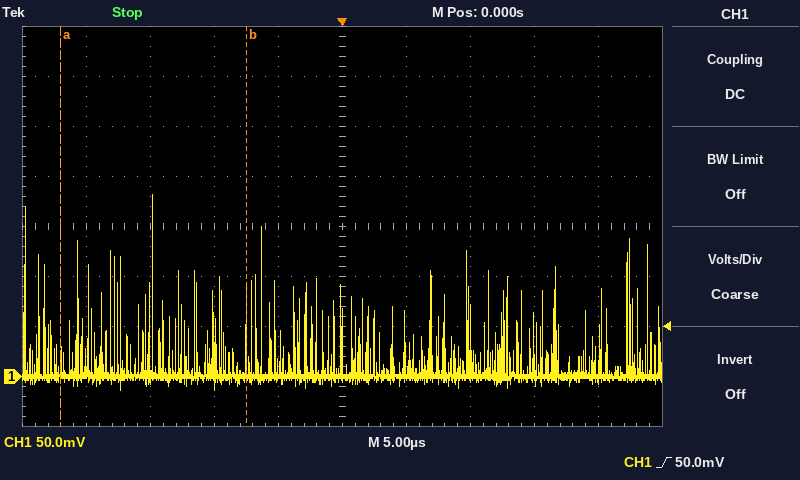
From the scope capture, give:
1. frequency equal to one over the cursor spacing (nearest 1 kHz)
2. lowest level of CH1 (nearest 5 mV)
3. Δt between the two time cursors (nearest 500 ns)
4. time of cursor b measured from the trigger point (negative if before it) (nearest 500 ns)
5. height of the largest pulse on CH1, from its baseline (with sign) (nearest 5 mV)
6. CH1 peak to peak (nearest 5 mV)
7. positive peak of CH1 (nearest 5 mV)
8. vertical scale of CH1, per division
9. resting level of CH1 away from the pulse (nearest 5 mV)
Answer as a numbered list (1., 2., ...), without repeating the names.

1. 69 kHz
2. -15 mV
3. 14.5 µs
4. -7.5 µs
5. +180 mV
6. 195 mV
7. 180 mV
8. 50 mV
9. 0 mV
